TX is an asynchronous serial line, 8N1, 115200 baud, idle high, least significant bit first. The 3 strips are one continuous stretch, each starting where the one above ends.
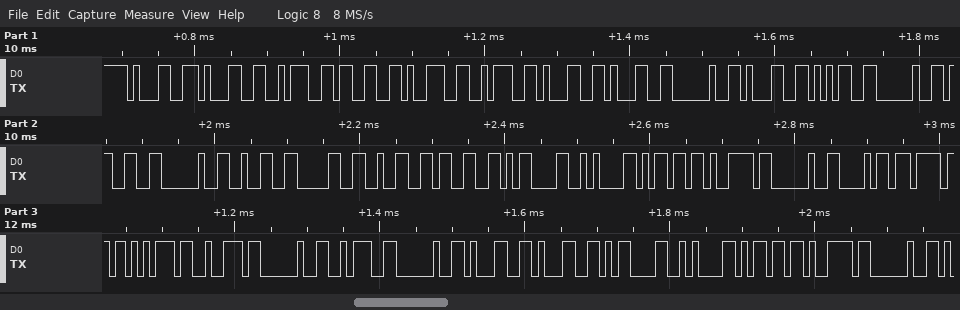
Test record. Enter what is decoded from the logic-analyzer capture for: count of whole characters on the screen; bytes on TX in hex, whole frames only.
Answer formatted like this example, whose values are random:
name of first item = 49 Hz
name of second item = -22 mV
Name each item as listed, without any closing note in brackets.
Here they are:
count of whole characters on the screen = 37
bytes on TX in hex, whole frames only = 0x31 0x31 0x3A 0x33 0x39 0x3A 0x31 0x31 0x20 0x31 0x35 0x20 0x33 0x20 0x32 0x30 0x32 0x33 0x0D 0x0A 0x6D 0x79 0x20 0x68 0x6F 0x75 0x72 0x20 0x3A 0x20 0x31 0x31 0x0D 0x0A 0x6D 0x79 0x20
